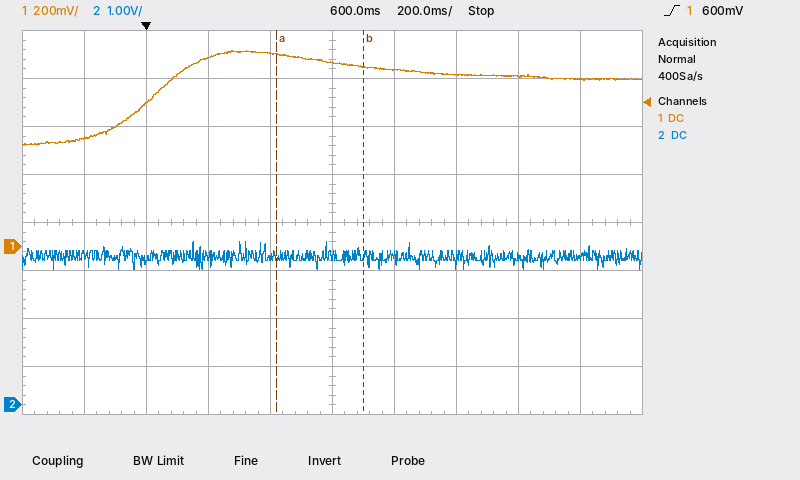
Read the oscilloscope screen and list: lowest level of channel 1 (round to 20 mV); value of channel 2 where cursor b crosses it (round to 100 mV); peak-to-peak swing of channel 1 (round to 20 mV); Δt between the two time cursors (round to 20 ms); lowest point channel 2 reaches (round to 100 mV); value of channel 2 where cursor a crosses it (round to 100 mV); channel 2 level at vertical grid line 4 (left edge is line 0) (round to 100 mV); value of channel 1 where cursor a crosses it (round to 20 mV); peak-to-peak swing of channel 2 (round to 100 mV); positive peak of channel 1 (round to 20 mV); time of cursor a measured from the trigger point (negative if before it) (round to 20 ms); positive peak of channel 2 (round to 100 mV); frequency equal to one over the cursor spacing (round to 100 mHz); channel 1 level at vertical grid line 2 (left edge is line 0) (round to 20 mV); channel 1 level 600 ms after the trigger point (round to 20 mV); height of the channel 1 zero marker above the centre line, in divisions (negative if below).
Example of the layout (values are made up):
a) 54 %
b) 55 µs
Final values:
a) 420 mV
b) 3.1 V
c) 400 mV
d) 280 ms
e) 2.8 V
f) 3.1 V
g) 3.1 V
h) 800 mV
i) 600 mV
j) 820 mV
k) +420 ms
l) 3.4 V
m) 3.6 Hz
n) 600 mV
o) 760 mV
p) -0.5 div
